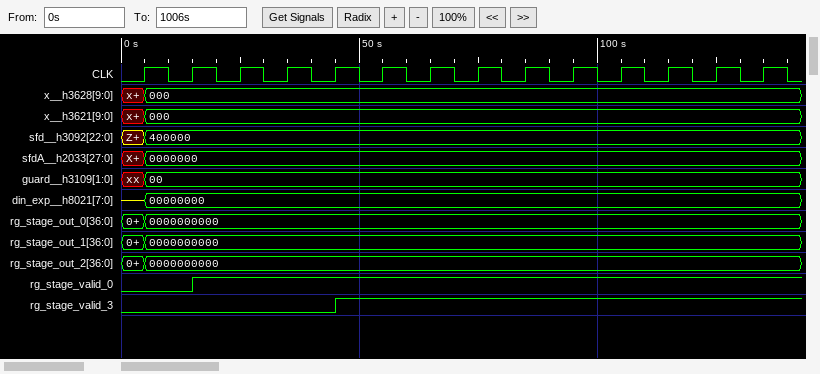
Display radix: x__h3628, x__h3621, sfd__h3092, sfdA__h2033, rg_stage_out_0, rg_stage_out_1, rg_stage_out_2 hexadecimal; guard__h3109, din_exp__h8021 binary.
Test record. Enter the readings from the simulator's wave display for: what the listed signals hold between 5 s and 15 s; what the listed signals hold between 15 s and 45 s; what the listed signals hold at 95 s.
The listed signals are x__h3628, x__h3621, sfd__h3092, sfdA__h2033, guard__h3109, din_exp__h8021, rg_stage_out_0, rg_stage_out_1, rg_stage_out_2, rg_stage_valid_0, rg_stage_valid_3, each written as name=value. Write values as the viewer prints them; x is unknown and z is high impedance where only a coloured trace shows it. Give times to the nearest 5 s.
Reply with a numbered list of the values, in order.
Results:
1. x__h3628=000, x__h3621=000, sfd__h3092=400000, sfdA__h2033=0000000, guard__h3109=00, din_exp__h8021=00000000, rg_stage_out_0=0000000000, rg_stage_out_1=0000000000, rg_stage_out_2=0000000000, rg_stage_valid_0=0, rg_stage_valid_3=0
2. x__h3628=000, x__h3621=000, sfd__h3092=400000, sfdA__h2033=0000000, guard__h3109=00, din_exp__h8021=00000000, rg_stage_out_0=0000000000, rg_stage_out_1=0000000000, rg_stage_out_2=0000000000, rg_stage_valid_0=1, rg_stage_valid_3=0
3. x__h3628=000, x__h3621=000, sfd__h3092=400000, sfdA__h2033=0000000, guard__h3109=00, din_exp__h8021=00000000, rg_stage_out_0=0000000000, rg_stage_out_1=0000000000, rg_stage_out_2=0000000000, rg_stage_valid_0=1, rg_stage_valid_3=1
